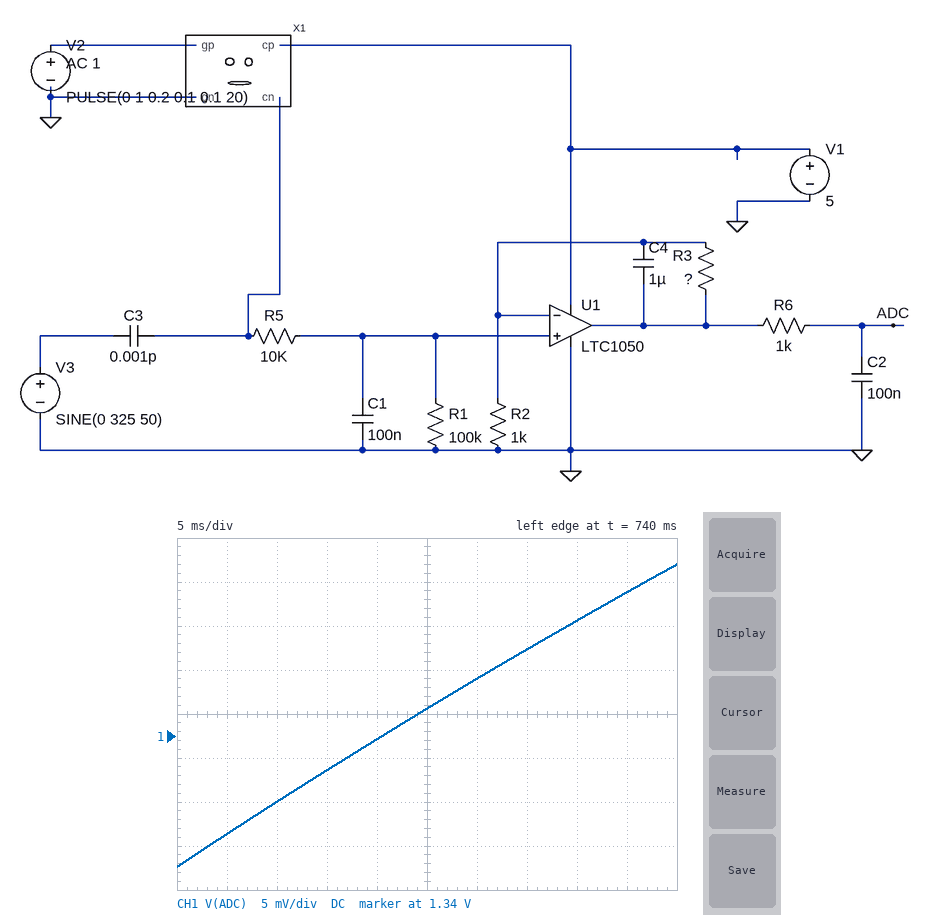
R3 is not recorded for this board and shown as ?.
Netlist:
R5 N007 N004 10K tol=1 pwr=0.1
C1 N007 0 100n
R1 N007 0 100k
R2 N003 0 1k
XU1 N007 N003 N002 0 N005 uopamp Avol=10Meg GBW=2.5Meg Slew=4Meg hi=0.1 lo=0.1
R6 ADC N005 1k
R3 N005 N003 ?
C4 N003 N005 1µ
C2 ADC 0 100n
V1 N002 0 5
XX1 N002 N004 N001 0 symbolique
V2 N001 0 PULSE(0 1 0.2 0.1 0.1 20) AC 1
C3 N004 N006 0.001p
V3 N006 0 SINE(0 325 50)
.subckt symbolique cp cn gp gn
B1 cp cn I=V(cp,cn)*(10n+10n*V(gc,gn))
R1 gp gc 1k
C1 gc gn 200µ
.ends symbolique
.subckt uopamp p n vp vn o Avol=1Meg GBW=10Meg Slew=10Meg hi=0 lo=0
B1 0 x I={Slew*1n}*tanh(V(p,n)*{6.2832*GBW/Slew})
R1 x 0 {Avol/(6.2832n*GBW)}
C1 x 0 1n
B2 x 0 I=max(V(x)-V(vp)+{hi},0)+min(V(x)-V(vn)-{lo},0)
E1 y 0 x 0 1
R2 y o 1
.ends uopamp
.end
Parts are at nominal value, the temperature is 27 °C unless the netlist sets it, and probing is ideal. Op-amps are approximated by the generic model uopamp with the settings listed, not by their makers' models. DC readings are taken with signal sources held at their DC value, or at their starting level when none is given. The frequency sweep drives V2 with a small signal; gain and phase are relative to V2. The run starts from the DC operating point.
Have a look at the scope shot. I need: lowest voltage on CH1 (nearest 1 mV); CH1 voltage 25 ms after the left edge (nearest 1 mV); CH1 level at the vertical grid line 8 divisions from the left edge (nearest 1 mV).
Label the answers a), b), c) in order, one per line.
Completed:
a) 1.325 V
b) 1.343 V
c) 1.353 V
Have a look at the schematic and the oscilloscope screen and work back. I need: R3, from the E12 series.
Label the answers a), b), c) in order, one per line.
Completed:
a) 150 kΩ
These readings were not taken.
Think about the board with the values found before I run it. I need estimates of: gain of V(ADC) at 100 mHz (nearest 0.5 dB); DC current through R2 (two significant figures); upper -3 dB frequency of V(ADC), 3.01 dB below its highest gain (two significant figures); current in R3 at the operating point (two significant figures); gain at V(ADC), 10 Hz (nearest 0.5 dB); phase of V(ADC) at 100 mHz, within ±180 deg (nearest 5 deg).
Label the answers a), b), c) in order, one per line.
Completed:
a) -2.5 dB
b) 5.0 µA
c) 580 mHz
d) 5.0 µA
e) -45.5 dB
f) -15 deg
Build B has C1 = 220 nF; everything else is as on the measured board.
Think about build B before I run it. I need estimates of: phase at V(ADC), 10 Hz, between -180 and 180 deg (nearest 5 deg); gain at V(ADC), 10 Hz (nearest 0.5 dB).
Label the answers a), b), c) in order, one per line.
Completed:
a) 140 deg
b) -48.5 dB
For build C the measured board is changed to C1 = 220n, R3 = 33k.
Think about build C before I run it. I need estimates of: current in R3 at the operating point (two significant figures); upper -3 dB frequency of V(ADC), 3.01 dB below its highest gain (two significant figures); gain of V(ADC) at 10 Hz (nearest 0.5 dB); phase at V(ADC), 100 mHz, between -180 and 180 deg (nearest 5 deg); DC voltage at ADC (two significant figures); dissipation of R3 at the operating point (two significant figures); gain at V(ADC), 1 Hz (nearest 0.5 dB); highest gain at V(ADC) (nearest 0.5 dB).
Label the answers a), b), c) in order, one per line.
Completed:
a) 5.0 µA
b) 770 mHz
c) -49.5 dB
d) -10 deg
e) 170 mV
f) 820 nW
g) -20.0 dB
h) -15.5 dB
